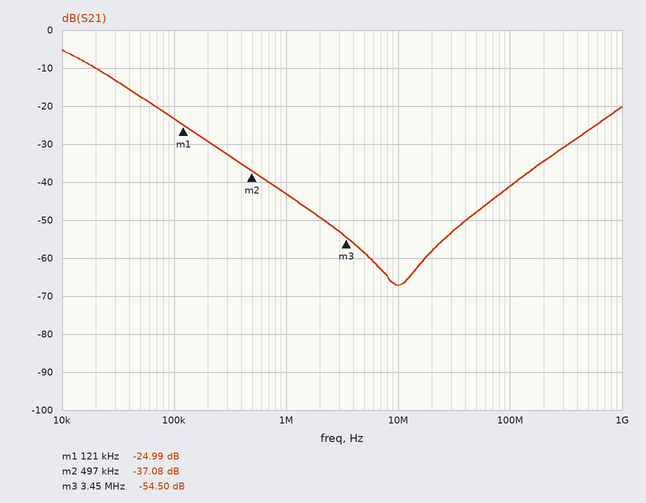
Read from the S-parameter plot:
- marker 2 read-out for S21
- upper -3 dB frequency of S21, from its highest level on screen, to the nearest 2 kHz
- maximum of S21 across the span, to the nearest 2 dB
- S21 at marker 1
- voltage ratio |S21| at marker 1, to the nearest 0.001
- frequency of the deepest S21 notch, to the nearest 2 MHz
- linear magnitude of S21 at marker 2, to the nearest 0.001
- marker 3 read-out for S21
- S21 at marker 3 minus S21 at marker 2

-37.08 dB
16 kHz
-6 dB
-24.99 dB
0.056
10 MHz
0.014
-54.50 dB
-17.42 dB
